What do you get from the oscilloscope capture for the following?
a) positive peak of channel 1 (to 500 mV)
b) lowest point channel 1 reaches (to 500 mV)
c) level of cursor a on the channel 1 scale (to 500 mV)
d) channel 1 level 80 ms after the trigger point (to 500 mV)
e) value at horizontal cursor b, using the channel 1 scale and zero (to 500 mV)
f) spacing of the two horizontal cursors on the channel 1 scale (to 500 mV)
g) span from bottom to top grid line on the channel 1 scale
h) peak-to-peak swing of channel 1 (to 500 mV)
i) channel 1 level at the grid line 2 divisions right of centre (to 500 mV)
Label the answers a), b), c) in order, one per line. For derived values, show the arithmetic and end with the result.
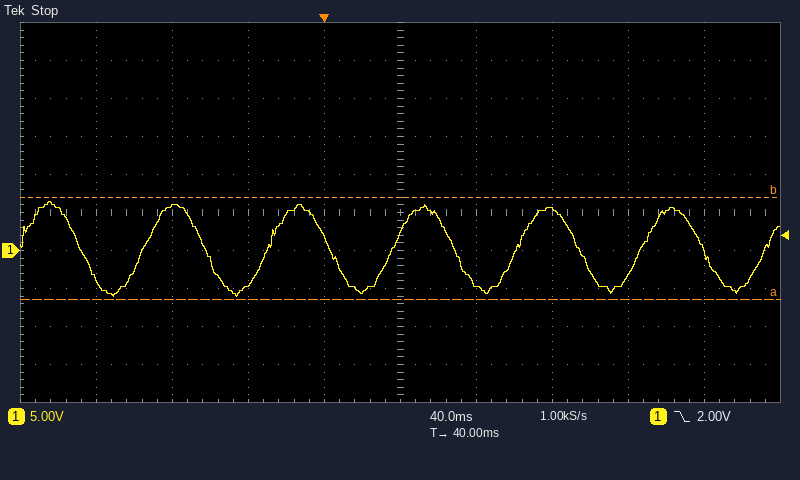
a) 6.5 V
b) -6.0 V
c) -6.5 V
d) -4.5 V
e) 7.0 V
f) 13.5 V
g) 50 V
h) 6.5 V − (-6.0 V) = 12.5 V
i) 5.5 V
